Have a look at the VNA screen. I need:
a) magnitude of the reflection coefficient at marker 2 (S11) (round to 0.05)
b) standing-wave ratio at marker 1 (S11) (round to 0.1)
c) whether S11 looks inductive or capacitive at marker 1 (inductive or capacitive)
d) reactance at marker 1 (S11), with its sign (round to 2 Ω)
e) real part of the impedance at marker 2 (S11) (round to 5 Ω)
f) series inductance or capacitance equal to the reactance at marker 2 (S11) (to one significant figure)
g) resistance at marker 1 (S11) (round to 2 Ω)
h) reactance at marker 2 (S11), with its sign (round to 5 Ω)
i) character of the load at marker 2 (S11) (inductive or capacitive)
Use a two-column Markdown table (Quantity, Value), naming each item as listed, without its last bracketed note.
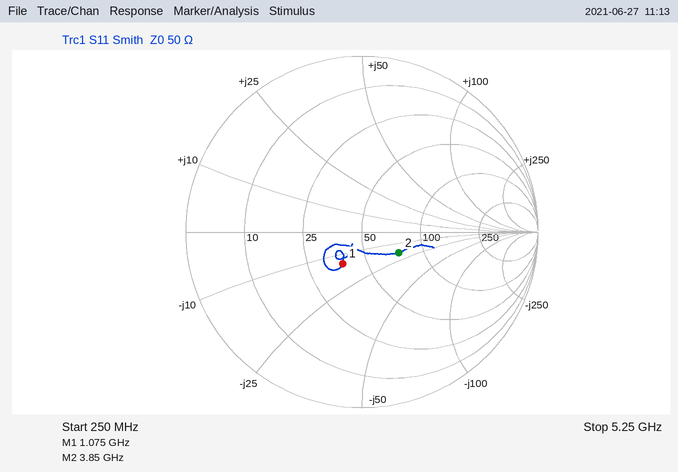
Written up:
| Quantity | Value |
|---|---|
| magnitude of the reflection coefficient at marker 2 (S11) | 0.25 |
| standing-wave ratio at marker 1 (S11) | 1.5 |
| whether S11 looks inductive or capacitive at marker 1 | capacitive |
| reactance at marker 1 (S11), with its sign | -14 Ω |
| real part of the impedance at marker 2 (S11) | 75 Ω |
| series inductance or capacitance equal to the reactance at marker 2 (S11) | 2 pF |
| resistance at marker 1 (S11) | 38 Ω |
| reactance at marker 2 (S11), with its sign | -20 Ω |
| character of the load at marker 2 (S11) | capacitive |
